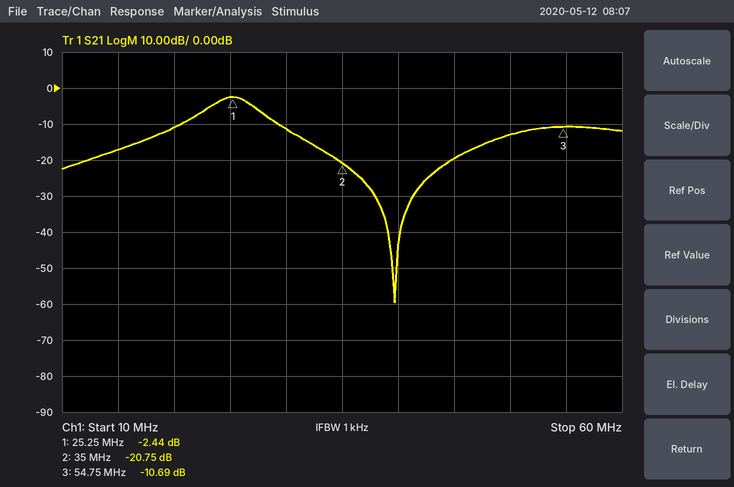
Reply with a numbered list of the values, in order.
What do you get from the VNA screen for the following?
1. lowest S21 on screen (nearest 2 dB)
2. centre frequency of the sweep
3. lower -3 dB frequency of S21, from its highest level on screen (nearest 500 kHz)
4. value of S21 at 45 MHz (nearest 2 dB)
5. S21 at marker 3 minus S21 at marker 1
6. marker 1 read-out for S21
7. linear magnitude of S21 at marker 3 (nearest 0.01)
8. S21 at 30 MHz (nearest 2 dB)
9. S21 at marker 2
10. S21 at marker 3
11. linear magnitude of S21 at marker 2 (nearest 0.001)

1. -60 dB
2. 35 MHz
3. 23.0 MHz
4. -20 dB
5. -8.25 dB
6. -2.44 dB
7. 0.29
8. -12 dB
9. -20.75 dB
10. -10.69 dB
11. 0.092
